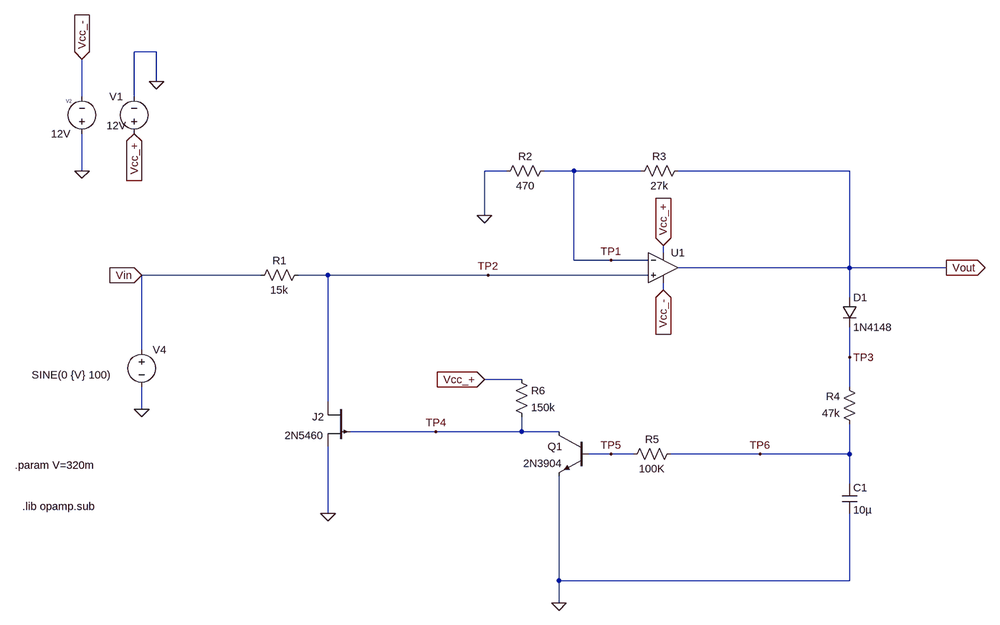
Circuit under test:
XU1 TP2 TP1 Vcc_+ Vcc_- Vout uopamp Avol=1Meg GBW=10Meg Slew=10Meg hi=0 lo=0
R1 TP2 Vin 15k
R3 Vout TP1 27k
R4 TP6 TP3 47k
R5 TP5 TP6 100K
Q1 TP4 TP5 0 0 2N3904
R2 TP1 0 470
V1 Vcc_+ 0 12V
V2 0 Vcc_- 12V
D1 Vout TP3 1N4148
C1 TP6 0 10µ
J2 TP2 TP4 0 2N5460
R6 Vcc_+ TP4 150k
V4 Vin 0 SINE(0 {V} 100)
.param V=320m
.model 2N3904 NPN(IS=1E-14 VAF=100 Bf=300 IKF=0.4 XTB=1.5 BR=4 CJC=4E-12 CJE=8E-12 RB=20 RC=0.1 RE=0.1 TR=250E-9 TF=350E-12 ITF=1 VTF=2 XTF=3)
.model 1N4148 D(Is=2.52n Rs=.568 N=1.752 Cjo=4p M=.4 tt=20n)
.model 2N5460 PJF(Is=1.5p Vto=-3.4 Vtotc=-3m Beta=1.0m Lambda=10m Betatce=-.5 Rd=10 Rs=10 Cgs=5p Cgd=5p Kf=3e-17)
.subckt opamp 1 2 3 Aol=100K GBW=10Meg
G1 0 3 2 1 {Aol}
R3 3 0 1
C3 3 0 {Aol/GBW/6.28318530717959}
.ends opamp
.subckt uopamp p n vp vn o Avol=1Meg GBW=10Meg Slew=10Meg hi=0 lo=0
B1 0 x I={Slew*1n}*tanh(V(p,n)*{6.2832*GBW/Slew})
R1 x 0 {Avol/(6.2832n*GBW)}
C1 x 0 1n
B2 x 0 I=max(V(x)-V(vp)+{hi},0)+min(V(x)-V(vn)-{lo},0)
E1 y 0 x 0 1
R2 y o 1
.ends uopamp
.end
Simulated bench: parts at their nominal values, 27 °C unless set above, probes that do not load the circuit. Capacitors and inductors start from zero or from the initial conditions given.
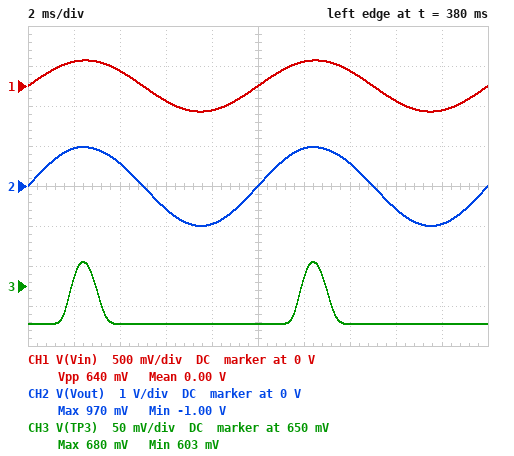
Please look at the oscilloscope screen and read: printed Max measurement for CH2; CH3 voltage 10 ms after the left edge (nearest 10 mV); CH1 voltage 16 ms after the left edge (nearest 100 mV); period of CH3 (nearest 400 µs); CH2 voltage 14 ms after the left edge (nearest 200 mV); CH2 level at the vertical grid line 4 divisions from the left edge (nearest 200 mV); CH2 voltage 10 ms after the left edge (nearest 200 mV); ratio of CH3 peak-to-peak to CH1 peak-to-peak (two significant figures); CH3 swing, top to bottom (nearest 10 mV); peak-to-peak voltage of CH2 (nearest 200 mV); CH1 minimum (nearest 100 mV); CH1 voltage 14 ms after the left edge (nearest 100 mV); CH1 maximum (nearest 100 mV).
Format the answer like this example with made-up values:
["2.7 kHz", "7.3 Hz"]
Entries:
["970 mV", "600 mV", "-200 mV", "10.0 ms", "600 mV", "-1.0 V", "0 V", "0.12", "80 mV", "2.0 V", "-300 mV", "200 mV", "300 mV"]
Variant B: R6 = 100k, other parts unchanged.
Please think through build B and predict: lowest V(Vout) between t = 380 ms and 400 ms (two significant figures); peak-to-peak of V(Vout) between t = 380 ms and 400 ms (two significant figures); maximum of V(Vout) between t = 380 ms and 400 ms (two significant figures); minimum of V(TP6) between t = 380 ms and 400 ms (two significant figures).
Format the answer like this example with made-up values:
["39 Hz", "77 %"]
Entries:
["-1.1 V", "2.1 V", "1.0 V", "620 mV"]
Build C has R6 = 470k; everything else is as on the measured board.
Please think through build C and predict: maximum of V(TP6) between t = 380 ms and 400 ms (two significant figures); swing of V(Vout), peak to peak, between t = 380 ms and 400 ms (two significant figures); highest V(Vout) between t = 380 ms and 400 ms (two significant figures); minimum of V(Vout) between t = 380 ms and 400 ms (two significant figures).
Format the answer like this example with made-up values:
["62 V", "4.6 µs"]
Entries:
["560 mV", "1.7 V", "840 mV", "-850 mV"]
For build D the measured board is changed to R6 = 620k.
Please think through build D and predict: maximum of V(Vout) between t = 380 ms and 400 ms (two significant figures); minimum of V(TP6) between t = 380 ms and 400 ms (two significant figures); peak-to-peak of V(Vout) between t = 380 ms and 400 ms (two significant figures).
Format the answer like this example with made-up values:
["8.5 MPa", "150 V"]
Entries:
["810 mV", "550 mV", "1.6 V"]
